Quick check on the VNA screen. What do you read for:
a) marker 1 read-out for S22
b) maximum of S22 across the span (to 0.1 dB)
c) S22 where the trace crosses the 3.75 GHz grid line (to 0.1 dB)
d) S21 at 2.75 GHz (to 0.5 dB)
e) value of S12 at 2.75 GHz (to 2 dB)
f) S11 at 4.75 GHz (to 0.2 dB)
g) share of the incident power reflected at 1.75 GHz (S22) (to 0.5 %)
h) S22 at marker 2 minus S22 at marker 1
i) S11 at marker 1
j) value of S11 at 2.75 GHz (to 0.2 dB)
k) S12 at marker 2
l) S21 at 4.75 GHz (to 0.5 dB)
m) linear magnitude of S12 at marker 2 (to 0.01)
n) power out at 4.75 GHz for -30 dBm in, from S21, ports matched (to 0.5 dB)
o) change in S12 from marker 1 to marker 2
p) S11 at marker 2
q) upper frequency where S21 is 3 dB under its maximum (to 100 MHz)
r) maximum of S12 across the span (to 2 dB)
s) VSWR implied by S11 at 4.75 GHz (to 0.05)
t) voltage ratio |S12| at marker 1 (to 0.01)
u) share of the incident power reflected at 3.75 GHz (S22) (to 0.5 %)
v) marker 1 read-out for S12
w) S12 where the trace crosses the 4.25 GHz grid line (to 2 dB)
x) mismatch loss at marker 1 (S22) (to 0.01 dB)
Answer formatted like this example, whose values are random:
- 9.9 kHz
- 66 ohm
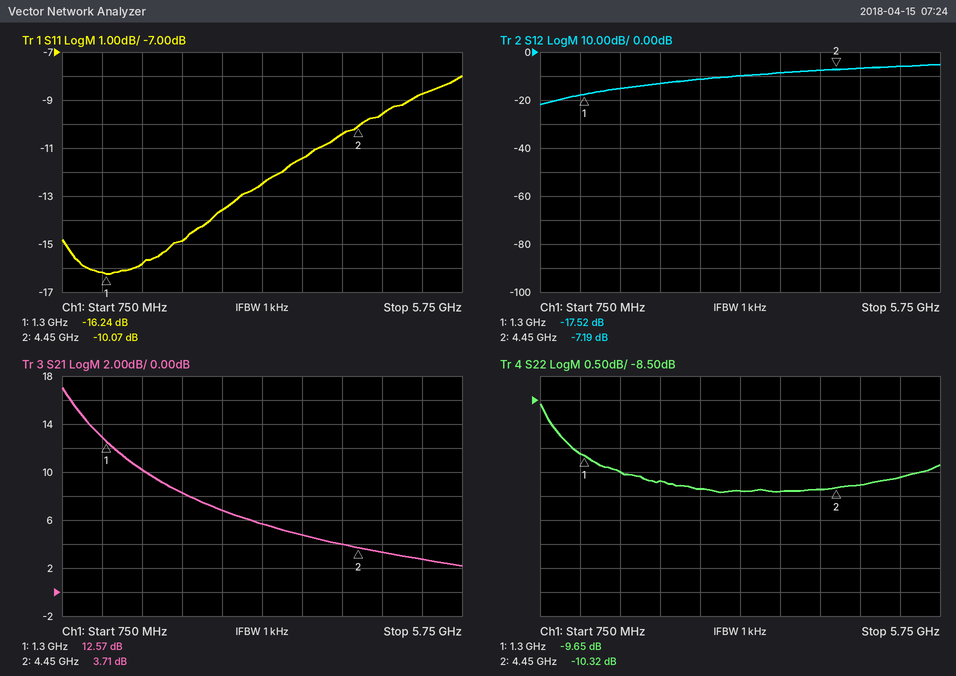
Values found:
- -9.65 dB
- -8.6 dB
- -10.4 dB
- 7.0 dB
- -12 dB
- -9.6 dB
- 10.0 %
- -0.67 dB
- -16.24 dB
- -13.6 dB
- -7.19 dB
- 3.5 dB
- 0.44
- -26.5 dBm
- 10.33 dB
- -10.07 dB
- 1.1 GHz
- -6 dB
- 2.00
- 0.13
- 9.0 %
- -17.52 dB
- -8 dB
- 0.50 dB
